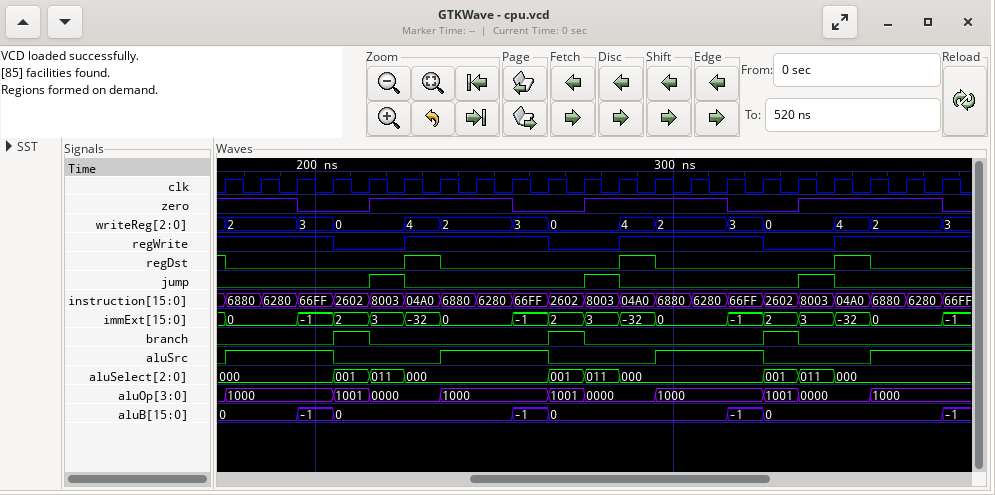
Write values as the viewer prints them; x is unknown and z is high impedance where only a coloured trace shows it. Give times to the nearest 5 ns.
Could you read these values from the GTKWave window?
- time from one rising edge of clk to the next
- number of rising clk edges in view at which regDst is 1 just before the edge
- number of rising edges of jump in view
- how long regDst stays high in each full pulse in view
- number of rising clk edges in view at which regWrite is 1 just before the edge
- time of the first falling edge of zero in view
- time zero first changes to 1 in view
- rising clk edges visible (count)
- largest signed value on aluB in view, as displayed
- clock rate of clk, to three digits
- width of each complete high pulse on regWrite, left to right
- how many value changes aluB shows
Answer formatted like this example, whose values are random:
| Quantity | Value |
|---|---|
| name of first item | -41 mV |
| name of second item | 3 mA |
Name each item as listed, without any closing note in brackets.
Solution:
| Quantity | Value |
|---|---|
| time from one rising edge of clk to the next | 10 ns |
| number of rising clk edges in view at which regDst is 1 just before the edge | 4 |
| number of rising edges of jump in view | 3 |
| how long regDst stays high in each full pulse in view | 10 ns, 10 ns, 10 ns |
| number of rising clk edges in view at which regWrite is 1 just before the edge | 15 |
| time of the first falling edge of zero in view | 195 ns |
| time zero first changes to 1 in view | 215 ns |
| rising clk edges visible | 21 |
| largest signed value on aluB in view, as displayed | 0 |
| clock rate of clk, to three digits | 100 MHz |
| width of each complete high pulse on regWrite, left to right | 40 ns, 40 ns |
| how many value changes aluB shows | 7 |
